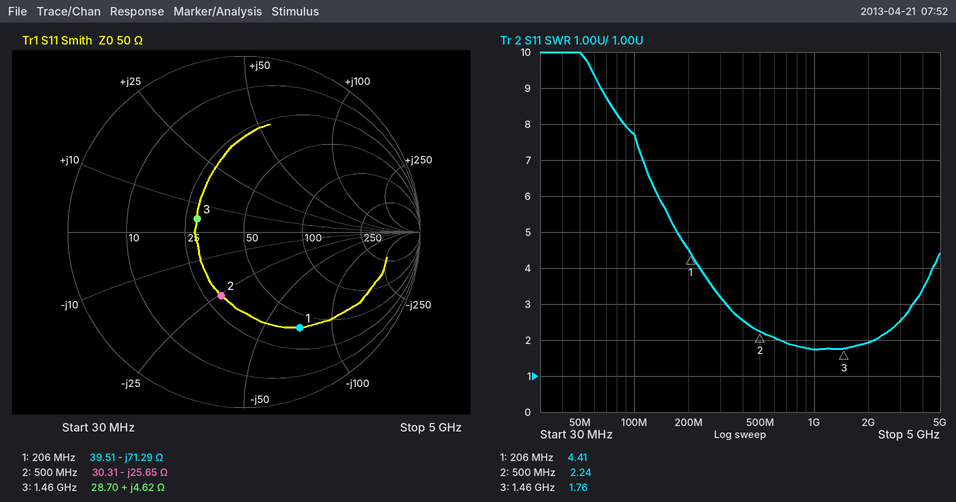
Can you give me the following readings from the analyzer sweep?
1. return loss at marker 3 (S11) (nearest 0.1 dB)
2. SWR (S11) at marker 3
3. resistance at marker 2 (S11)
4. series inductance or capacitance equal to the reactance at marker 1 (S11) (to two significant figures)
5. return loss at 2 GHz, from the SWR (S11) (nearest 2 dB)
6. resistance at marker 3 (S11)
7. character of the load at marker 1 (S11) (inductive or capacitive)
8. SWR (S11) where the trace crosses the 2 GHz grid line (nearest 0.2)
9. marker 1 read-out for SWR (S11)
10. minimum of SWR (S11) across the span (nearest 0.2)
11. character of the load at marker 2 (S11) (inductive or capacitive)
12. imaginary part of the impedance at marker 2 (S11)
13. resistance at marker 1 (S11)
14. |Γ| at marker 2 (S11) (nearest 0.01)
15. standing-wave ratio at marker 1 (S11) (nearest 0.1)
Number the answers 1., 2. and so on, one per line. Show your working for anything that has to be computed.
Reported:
1. 11.2 dB
2. 1.76
3. 30.31 Ω
4. C = 1/(2π × 206 MHz × 71.29 Ω) ≈ 11 pF
5. −20 log10((2 − 1)/(2 + 1)) ≈ 10 dB
6. 28.70 Ω
7. capacitive
8. 2.0
9. 4.41
10. 1.8
11. capacitive
12. -25.65 Ω
13. 39.51 Ω
14. 0.38
15. 4.4
